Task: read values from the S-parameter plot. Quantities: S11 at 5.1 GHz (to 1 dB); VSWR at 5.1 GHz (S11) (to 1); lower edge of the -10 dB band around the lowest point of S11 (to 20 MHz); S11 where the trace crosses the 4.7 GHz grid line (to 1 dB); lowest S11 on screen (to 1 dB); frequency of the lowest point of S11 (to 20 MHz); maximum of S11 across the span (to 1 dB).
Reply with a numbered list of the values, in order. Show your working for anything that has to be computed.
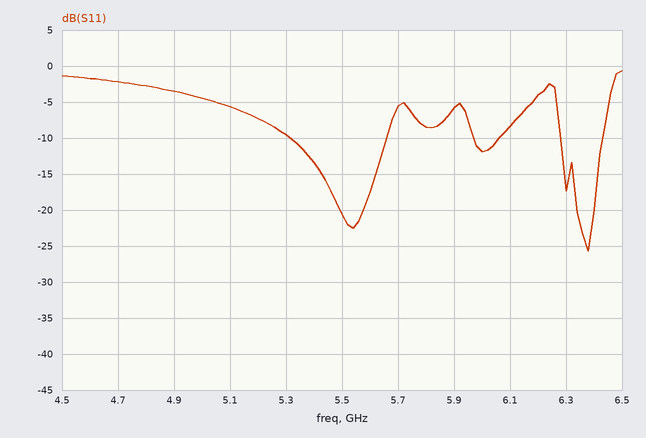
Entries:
1. -6 dB
2. |Γ| = 10^(-6/20) = 0.5012; VSWR = (1 + 0.5012)/(1 − 0.5012) ≈ 3
3. 6.28 GHz
4. -2 dB
5. -26 dB
6. 6.38 GHz
7. -1 dB
